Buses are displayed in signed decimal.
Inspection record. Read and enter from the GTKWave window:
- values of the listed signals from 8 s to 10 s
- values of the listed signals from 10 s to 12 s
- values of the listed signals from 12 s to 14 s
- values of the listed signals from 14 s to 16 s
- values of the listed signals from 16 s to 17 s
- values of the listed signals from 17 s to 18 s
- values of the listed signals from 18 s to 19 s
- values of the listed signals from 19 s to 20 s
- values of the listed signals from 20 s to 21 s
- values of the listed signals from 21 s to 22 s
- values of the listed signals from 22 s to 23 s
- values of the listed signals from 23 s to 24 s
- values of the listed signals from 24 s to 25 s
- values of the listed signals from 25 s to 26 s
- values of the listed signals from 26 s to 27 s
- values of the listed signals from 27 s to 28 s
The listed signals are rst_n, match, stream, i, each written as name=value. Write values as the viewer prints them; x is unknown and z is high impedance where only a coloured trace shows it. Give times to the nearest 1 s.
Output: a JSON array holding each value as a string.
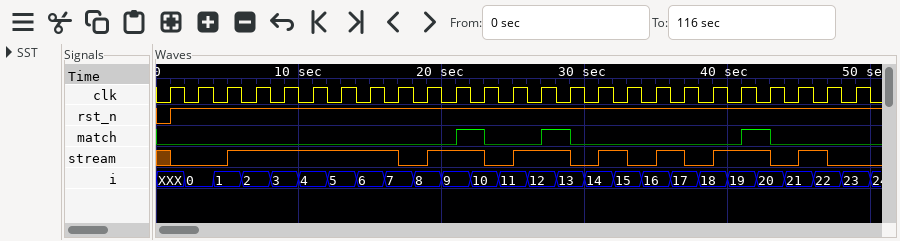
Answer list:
["rst_n=1, match=0, stream=1, i=3", "rst_n=1, match=0, stream=1, i=4", "rst_n=1, match=0, stream=1, i=5", "rst_n=1, match=0, stream=1, i=6", "rst_n=1, match=0, stream=1, i=7", "rst_n=1, match=0, stream=0, i=7", "rst_n=1, match=0, stream=0, i=8", "rst_n=1, match=0, stream=1, i=8", "rst_n=1, match=0, stream=1, i=9", "rst_n=1, match=1, stream=1, i=9", "rst_n=1, match=1, stream=1, i=10", "rst_n=1, match=0, stream=0, i=10", "rst_n=1, match=0, stream=0, i=11", "rst_n=1, match=0, stream=1, i=11", "rst_n=1, match=0, stream=1, i=12", "rst_n=1, match=1, stream=1, i=12"]
